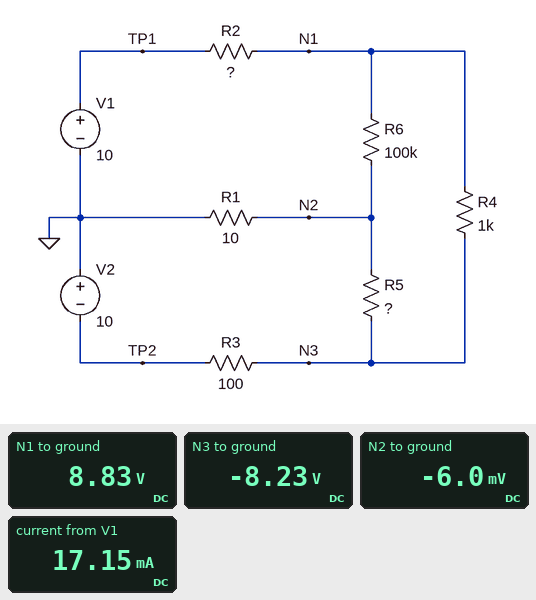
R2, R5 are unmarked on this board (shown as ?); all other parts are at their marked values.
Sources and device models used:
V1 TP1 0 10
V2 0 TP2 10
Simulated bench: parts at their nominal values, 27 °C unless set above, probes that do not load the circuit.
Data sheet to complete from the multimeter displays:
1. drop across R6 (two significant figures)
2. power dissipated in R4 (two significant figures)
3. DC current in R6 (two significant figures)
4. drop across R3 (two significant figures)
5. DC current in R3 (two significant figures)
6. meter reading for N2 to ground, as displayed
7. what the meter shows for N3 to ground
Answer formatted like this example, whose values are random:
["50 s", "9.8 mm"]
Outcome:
["8.8 V", "290 mW", "88 µA", "1.8 V", "18 mA", "-6.0 mV", "-8.23 V"]
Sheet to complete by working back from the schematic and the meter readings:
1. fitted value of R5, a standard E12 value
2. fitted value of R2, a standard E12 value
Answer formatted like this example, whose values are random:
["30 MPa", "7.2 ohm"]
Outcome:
["12 kΩ", "68 Ω"]
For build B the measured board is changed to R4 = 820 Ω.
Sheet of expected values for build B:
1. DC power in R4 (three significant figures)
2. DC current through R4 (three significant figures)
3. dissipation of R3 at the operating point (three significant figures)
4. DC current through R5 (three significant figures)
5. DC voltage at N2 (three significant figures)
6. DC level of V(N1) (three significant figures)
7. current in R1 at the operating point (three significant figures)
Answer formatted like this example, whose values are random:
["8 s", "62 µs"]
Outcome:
["334 mW", "20.2 mA", "43.4 mW", "659 µA", "-5.73 mV", "8.62 V", "573 µA"]
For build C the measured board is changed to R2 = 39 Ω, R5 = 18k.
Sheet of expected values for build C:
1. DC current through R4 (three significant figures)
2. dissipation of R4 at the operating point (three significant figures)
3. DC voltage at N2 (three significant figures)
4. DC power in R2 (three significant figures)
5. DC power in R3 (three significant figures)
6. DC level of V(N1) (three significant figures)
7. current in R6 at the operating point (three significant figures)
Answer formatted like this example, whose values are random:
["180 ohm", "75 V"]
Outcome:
["17.5 mA", "307 mW", "-3.62 mV", "12.1 mW", "32.3 mW", "9.31 V", "93.2 µA"]
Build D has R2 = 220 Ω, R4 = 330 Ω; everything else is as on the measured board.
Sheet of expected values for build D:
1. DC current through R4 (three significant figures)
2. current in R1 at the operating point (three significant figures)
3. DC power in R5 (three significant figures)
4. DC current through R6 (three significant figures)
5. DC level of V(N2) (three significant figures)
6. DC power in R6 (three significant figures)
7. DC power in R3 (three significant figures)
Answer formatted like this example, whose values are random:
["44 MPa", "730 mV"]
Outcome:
["30.7 mA", "540 µA", "3.93 mW", "32.5 µA", "-5.40 mV", "106 µW", "97.6 mW"]
